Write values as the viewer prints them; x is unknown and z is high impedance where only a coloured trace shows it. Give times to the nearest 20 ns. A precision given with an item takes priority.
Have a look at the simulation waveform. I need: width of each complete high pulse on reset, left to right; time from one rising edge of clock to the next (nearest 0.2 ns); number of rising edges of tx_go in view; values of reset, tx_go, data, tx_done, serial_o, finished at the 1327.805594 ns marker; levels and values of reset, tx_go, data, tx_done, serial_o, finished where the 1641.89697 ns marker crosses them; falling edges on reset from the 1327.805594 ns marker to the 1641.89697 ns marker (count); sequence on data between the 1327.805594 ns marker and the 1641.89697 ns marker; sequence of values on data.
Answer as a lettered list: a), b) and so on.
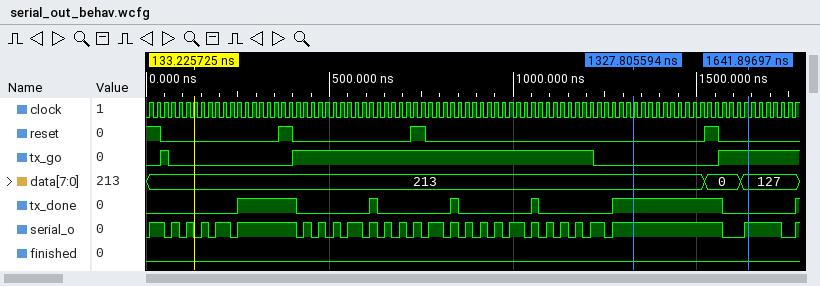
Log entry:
a) 40 ns, 40 ns, 40 ns
b) 20 ns
c) 3
d) reset=0, tx_go=0, data=213, tx_done=1, serial_o=1, finished=0
e) reset=0, tx_go=1, data=127, tx_done=0, serial_o=1, finished=0
f) 1
g) 213, 0, 127
h) 213, 0, 127
